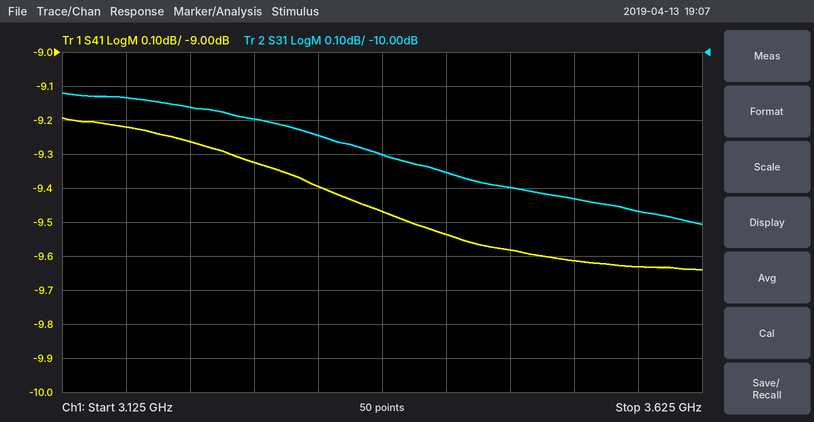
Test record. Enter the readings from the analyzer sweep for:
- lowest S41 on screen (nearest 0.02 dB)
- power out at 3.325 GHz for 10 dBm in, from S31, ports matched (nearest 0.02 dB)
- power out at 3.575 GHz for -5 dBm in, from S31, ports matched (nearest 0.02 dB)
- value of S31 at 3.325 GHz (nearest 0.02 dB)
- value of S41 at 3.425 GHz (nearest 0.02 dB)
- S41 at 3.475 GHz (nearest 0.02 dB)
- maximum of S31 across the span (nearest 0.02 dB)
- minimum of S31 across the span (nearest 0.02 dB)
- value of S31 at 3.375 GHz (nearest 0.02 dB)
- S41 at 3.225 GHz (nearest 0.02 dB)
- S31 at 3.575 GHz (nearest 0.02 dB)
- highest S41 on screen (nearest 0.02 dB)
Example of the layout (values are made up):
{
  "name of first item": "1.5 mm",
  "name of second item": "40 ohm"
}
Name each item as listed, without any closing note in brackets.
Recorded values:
{
  "lowest S41 on screen": "-9.64 dB",
  "power out at 3.325 GHz for 10 dBm in, from S31, ports matched": "-0.24 dBm",
  "power out at 3.575 GHz for -5 dBm in, from S31, ports matched": "-15.46 dBm",
  "value of S31 at 3.325 GHz": "-10.24 dB",
  "value of S41 at 3.425 GHz": "-9.54 dB",
  "S41 at 3.475 GHz": "-9.58 dB",
  "maximum of S31 across the span": "-10.12 dB",
  "minimum of S31 across the span": "-10.50 dB",
  "value of S31 at 3.375 GHz": "-10.30 dB",
  "S41 at 3.225 GHz": "-9.26 dB",
  "S31 at 3.575 GHz": "-10.46 dB",
  "highest S41 on screen": "-9.20 dB"
}
